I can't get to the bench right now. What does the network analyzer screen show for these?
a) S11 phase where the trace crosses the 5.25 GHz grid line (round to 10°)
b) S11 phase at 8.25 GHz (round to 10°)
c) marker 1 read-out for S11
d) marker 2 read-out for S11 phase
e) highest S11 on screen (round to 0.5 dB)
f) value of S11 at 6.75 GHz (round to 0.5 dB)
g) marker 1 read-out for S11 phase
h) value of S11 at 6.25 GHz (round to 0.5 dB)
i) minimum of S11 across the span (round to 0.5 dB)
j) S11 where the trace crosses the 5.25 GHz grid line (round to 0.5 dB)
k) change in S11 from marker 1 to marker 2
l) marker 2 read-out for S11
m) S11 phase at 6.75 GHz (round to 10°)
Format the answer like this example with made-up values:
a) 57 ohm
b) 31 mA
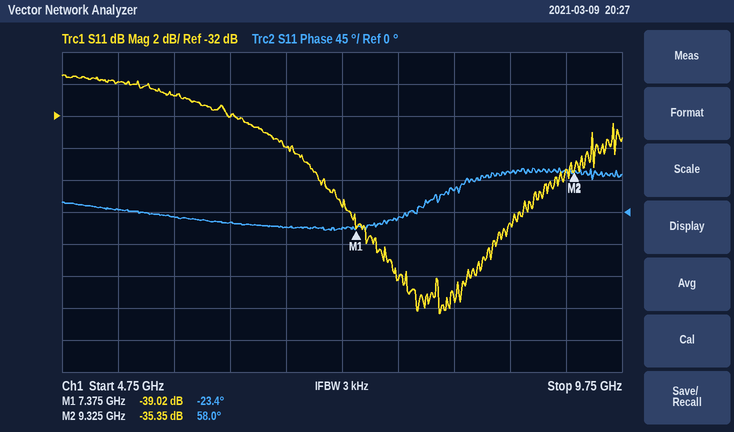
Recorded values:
a) 0°
b) 30°
c) -39.02 dB
d) 58.0°
e) -29.5 dB
f) -34.0 dB
g) -23.4°
h) -32.0 dB
i) -44.5 dB
j) -30.0 dB
k) 3.67 dB
l) -35.35 dB
m) -20°
